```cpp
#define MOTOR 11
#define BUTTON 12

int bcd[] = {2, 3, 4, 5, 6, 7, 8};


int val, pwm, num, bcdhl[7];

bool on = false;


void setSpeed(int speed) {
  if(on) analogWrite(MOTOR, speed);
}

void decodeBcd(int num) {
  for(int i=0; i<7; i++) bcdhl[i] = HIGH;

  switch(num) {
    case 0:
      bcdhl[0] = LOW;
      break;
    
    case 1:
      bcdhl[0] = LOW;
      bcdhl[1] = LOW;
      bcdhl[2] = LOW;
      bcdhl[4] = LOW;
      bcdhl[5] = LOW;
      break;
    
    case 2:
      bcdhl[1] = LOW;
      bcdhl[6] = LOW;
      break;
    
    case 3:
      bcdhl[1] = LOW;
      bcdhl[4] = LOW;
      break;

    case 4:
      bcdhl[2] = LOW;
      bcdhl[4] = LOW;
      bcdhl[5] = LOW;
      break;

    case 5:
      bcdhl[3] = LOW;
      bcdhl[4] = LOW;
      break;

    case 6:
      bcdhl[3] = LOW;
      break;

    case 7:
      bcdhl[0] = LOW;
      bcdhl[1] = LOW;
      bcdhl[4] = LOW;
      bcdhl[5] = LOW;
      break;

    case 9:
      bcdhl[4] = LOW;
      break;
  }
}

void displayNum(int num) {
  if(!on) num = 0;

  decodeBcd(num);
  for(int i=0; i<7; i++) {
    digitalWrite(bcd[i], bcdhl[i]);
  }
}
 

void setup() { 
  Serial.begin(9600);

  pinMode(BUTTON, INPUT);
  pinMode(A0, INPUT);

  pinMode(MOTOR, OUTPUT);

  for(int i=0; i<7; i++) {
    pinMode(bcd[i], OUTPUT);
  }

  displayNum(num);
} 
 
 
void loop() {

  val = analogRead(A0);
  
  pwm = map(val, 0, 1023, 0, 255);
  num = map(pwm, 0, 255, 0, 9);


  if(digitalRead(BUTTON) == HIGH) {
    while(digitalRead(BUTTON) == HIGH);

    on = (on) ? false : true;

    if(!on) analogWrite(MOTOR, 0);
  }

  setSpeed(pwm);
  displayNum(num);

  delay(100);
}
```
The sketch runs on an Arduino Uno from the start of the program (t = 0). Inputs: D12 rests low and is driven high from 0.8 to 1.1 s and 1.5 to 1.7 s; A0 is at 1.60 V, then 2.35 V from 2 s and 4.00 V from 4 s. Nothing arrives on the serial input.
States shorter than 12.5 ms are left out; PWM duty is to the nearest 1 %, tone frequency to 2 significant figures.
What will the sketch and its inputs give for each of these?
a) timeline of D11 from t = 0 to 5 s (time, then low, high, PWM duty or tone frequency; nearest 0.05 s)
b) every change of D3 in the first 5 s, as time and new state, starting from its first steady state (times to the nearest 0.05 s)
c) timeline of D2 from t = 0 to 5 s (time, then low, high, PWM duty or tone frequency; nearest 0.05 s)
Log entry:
0 s low; 1.1 s PWM 32 %; 1.7 s low
0 s high; 1.1 s low; 1.7 s high
0 s low; 1.1 s high; 1.7 s low
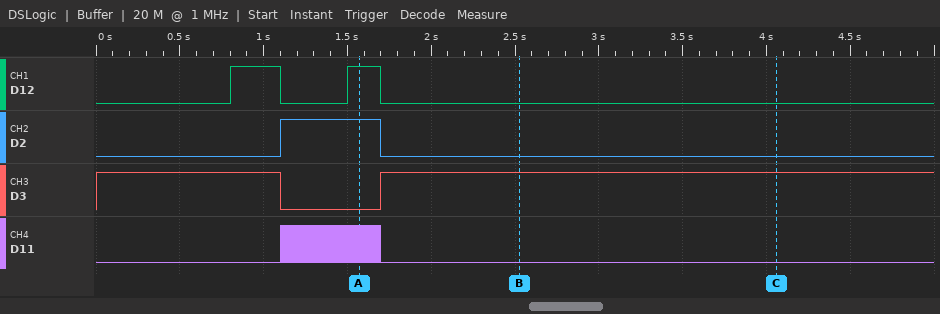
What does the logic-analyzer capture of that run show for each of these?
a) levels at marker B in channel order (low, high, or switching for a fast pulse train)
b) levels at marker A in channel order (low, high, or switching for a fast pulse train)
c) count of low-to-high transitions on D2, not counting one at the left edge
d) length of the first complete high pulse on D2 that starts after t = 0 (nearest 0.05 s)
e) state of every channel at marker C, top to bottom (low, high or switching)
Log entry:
D12 low, D2 low, D3 high, D11 low
D12 high, D2 high, D3 low, D11 switching
1
0.60 s
D12 low, D2 low, D3 high, D11 low
